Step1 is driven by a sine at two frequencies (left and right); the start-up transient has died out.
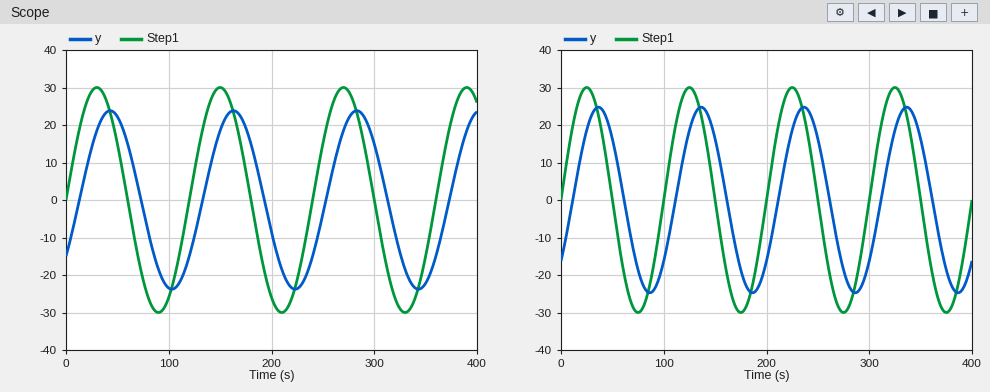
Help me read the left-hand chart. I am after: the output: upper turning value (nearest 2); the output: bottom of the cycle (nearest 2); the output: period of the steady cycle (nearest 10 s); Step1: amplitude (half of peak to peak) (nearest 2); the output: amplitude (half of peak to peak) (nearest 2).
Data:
24
-24
120 s
30
24
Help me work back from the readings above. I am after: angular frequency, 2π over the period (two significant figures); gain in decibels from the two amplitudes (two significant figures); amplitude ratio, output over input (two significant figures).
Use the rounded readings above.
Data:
0.052 rad/s
-1.9 dB
0.80
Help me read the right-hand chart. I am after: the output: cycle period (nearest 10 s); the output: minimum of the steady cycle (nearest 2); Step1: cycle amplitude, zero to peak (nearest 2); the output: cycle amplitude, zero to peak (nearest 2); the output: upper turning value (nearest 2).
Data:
100 s
-24
30
24
24
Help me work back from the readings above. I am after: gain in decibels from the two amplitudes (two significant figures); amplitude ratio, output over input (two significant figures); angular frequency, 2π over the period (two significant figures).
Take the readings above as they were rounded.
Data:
-1.9 dB
0.80
0.063 rad/s
